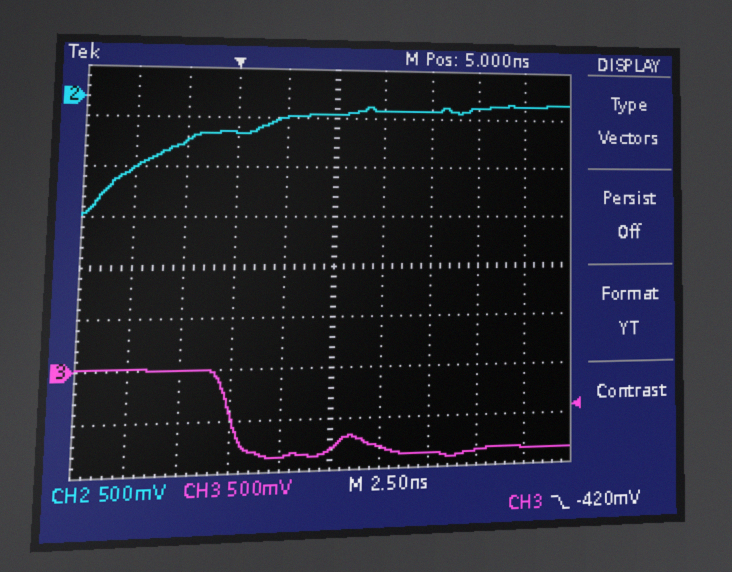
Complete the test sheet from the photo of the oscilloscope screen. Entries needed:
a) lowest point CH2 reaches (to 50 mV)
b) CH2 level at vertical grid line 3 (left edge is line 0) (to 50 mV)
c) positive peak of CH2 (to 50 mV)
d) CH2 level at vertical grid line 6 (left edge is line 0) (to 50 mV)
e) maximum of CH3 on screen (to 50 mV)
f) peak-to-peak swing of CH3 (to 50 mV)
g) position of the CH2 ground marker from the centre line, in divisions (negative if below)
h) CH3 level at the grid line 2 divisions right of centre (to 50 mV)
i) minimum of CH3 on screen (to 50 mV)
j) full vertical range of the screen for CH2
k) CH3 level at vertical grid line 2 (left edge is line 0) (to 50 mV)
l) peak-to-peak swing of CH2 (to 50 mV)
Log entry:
-1.20 V
-350 mV
-50 mV
-100 mV
0 mV
900 mV
+3.4 div
-850 mV
-900 mV
4 V
0 mV
1.15 V
